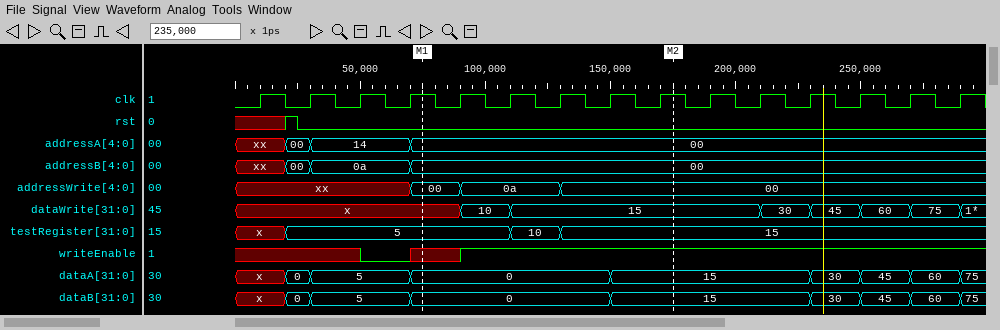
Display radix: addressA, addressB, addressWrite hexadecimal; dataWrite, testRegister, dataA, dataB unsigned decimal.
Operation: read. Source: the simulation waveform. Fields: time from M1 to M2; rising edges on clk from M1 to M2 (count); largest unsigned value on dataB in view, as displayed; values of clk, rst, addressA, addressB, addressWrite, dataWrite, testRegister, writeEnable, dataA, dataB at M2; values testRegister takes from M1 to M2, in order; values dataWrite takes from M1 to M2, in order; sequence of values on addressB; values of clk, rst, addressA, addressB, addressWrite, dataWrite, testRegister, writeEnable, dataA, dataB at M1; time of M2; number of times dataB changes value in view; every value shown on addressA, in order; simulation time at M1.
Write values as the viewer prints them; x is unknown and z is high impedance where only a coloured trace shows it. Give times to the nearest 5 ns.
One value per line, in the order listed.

100 ns
5
75
clk=1, rst=0, addressA=00, addressB=00, addressWrite=00, dataWrite=15, testRegister=15, writeEnable=1, dataA=15, dataB=15
5, 10, 15
x, 10, 15
xx, 00, 0a, 00
clk=1, rst=0, addressA=00, addressB=00, addressWrite=00, dataWrite=x, testRegister=5, writeEnable=x, dataA=0, dataB=0
175 ns
8
xx, 00, 14, 00
75 ns
